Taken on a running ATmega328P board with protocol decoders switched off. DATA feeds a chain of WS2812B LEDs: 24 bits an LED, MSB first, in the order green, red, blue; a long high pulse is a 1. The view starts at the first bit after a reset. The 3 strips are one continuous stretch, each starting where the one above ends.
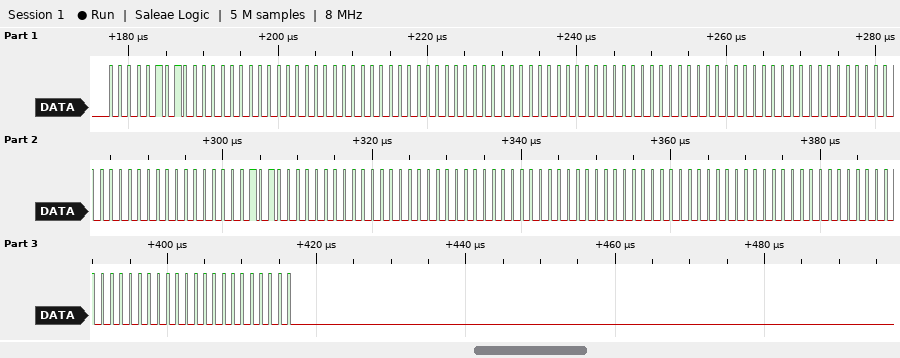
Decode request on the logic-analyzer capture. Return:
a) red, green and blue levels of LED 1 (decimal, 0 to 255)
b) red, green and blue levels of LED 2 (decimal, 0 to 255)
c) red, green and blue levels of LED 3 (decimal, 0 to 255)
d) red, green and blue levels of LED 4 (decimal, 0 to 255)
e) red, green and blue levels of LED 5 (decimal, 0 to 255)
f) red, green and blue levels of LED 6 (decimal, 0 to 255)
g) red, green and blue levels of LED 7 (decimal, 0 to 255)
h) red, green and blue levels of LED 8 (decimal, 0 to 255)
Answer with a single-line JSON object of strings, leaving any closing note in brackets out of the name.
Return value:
{"red, green and blue levels of LED 1": "0, 5, 0", "red, green and blue levels of LED 2": "0, 0, 0", "red, green and blue levels of LED 3": "0, 0, 0", "red, green and blue levels of LED 4": "0, 0, 0", "red, green and blue levels of LED 5": "0, 5, 0", "red, green and blue levels of LED 6": "0, 0, 0", "red, green and blue levels of LED 7": "0, 0, 0", "red, green and blue levels of LED 8": "0, 0, 0"}
